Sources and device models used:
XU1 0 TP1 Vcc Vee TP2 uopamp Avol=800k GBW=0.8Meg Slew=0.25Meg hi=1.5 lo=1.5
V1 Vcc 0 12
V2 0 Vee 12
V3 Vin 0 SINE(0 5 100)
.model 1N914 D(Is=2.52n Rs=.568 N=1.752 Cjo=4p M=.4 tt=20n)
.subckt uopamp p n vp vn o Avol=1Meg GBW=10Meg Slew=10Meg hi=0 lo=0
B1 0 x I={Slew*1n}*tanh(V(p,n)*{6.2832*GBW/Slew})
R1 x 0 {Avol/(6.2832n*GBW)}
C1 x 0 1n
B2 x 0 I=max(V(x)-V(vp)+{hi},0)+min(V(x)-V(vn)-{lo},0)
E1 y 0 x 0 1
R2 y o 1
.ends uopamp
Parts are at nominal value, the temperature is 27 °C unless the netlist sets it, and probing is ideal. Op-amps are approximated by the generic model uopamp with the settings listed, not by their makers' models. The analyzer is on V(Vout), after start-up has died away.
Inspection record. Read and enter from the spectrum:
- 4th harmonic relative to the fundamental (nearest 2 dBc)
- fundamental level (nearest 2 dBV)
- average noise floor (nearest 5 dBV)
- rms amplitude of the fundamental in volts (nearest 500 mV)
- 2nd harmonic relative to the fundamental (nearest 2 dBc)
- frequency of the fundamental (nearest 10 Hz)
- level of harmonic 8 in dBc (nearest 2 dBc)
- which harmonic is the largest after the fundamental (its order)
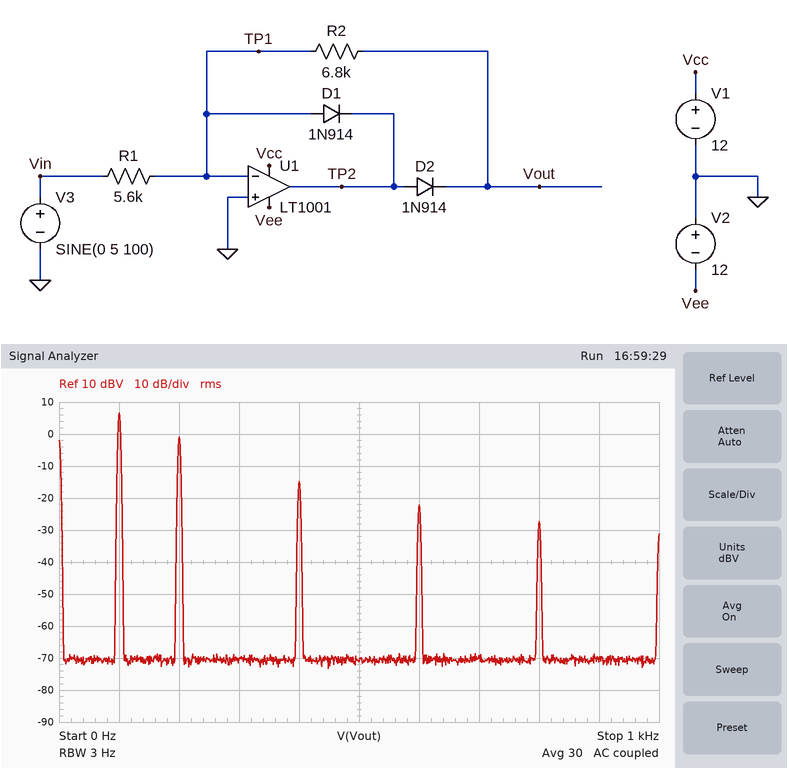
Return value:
-22 dBc
6 dBV
-70 dBV
2.0 V
-8 dBc
100 Hz
-34 dBc
2
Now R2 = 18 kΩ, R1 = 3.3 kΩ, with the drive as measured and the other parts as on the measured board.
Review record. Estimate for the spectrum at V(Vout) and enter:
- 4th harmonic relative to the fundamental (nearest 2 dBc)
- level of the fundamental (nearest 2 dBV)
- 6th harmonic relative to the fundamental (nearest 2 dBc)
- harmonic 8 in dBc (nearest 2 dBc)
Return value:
-16 dBc
12 dBV
-18 dBc
-22 dBc
